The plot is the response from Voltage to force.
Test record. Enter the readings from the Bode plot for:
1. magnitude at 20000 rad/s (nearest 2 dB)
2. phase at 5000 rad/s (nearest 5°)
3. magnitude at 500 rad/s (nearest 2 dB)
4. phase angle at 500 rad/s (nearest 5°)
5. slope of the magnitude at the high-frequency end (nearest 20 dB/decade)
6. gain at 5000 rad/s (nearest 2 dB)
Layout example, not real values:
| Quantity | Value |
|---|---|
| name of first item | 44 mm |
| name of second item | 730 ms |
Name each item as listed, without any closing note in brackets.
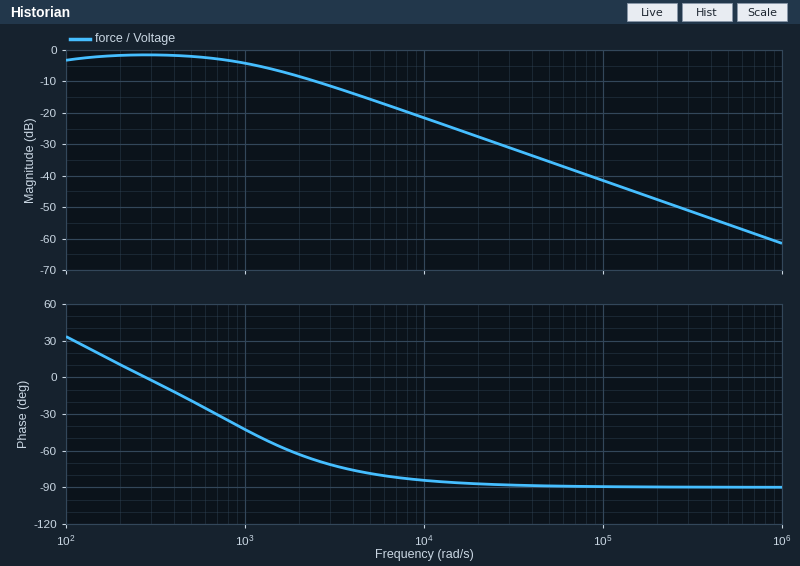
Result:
| Quantity | Value |
|---|---|
| magnitude at 20000 rad/s | -28 dB |
| phase at 5000 rad/s | -80° |
| magnitude at 500 rad/s | -2 dB |
| phase angle at 500 rad/s | -20° |
| slope of the magnitude at the high-frequency end | -20 dB/decade |
| gain at 5000 rad/s | -16 dB |
